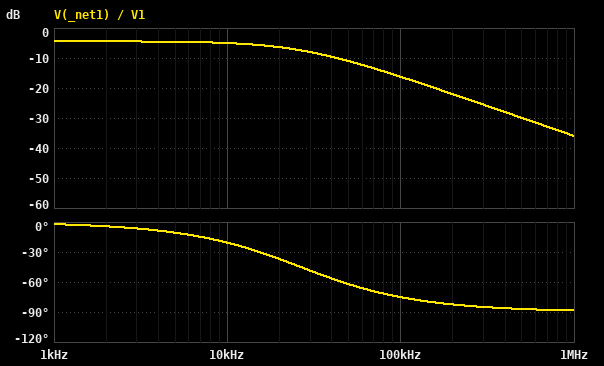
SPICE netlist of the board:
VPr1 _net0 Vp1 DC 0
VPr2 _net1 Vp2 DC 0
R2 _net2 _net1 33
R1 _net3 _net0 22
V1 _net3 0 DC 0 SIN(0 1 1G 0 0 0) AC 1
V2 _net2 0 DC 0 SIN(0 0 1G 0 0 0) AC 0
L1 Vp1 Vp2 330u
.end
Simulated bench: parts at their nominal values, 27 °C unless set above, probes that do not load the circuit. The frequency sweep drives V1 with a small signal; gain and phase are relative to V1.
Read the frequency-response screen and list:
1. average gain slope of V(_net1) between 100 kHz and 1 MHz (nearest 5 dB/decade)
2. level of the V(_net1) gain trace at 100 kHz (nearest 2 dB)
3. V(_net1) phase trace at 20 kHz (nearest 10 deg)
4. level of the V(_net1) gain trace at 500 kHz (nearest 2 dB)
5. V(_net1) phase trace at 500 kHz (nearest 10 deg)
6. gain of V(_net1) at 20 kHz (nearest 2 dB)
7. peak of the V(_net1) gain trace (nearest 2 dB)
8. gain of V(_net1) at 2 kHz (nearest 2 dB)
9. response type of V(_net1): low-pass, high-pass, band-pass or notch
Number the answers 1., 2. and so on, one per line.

1. -20 dB/decade
2. -16 dB
3. -40 deg
4. -30 dB
5. -90 deg
6. -6 dB
7. -4 dB
8. -4 dB
9. low-pass
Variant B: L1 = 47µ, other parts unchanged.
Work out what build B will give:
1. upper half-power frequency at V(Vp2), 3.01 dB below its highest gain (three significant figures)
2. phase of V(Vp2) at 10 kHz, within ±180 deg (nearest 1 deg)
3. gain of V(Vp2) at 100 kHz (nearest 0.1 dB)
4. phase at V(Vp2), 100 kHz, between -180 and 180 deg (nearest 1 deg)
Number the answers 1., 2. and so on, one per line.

1. 186 kHz
2. -3 deg
3. -5.5 dB
4. -28 deg
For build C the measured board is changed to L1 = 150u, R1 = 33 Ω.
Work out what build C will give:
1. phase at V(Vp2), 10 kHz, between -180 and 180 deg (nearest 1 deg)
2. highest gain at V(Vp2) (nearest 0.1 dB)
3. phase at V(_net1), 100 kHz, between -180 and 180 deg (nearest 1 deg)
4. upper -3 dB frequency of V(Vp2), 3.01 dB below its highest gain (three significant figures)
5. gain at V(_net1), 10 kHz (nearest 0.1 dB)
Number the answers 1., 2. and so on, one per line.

1. -8 deg
2. -6.0 dB
3. -55 deg
4. 70.0 kHz
5. -6.1 dB
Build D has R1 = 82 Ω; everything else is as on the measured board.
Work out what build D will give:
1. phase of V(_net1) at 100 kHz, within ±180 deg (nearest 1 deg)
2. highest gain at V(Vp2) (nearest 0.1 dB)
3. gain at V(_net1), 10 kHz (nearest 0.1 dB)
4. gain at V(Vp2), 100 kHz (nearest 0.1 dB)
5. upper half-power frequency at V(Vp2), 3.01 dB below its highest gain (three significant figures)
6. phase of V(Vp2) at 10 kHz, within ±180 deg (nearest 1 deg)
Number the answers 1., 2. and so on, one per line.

1. -61 deg
2. -10.8 dB
3. -11.0 dB
4. -17.1 dB
5. 55.5 kHz
6. -10 deg
